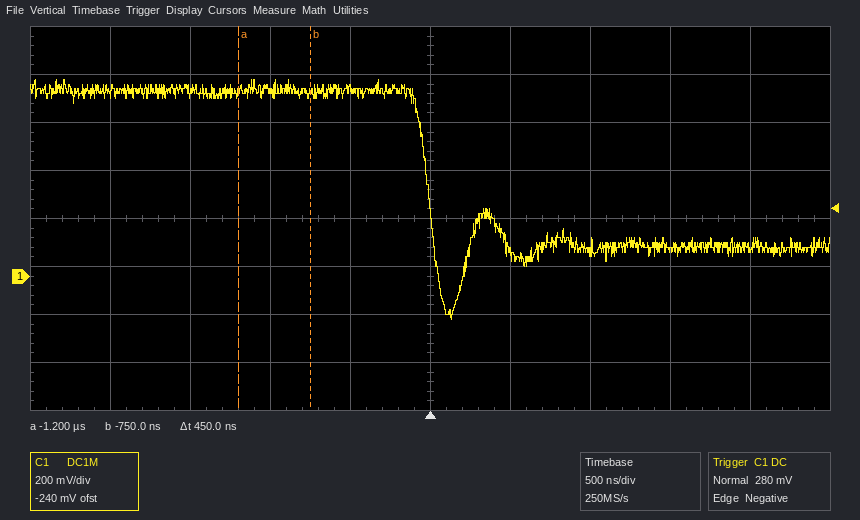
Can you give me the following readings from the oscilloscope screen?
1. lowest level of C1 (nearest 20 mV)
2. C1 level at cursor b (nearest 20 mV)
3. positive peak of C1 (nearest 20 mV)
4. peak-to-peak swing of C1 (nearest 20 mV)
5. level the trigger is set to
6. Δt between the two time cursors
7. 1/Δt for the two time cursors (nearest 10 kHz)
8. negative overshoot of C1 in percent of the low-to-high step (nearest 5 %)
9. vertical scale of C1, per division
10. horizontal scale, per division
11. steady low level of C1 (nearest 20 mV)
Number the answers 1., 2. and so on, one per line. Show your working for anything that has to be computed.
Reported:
1. -180 mV
2. 760 mV
3. 820 mV
4. 820 mV − (-180 mV) = 1.00 V
5. 280 mV
6. 450 ns
7. 1 / 450 ns ≈ 2.22 MHz
8. 45 %
9. 200 mV
10. 500 ns
11. 120 mV
